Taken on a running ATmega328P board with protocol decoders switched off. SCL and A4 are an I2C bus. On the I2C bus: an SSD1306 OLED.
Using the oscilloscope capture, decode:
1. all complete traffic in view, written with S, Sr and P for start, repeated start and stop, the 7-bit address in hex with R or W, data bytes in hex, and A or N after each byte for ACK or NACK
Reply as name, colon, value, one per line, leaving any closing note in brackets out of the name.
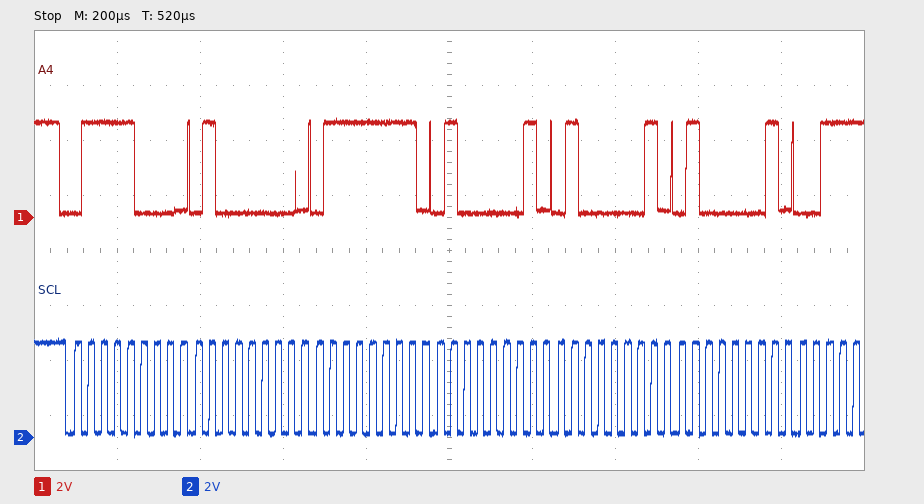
all complete traffic in view, written with S, Sr and P for start, repeated start and stop, the 7-bit address in hex with R or W, data bytes in hex, and A or N after each byte for ACK or NACK: S 3CW A 40 A 7F A 41 A 41 A 41 A
